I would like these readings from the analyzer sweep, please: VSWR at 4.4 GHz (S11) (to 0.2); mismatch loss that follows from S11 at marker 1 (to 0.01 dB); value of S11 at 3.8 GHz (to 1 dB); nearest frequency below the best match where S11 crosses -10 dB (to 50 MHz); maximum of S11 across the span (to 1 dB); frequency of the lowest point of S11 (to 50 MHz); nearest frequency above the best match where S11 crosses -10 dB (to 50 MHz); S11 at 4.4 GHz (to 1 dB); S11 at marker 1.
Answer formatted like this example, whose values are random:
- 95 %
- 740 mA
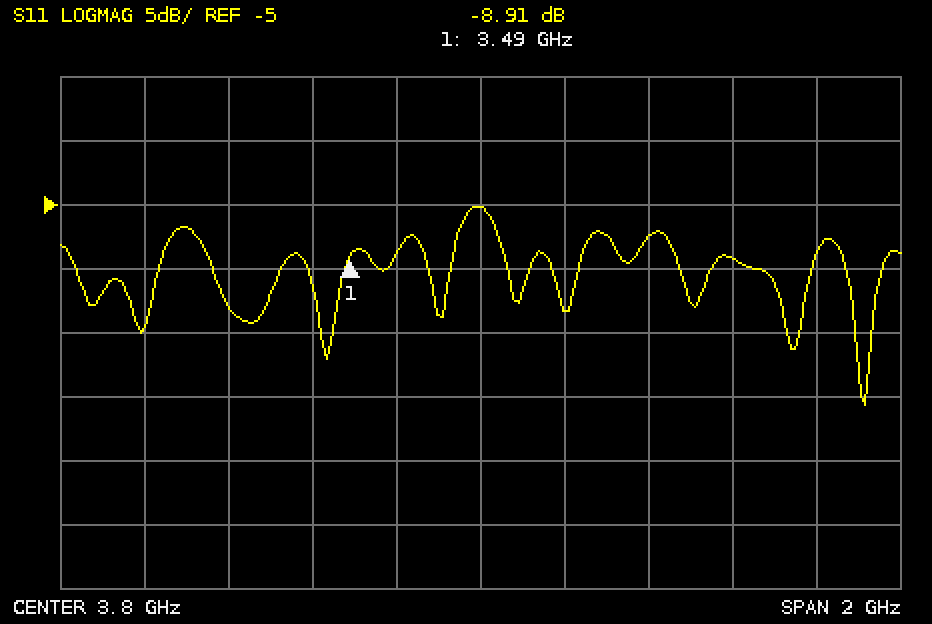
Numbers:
- 2.0
- 0.60 dB
- -5 dB
- 4.65 GHz
- -5 dB
- 4.70 GHz
- 4.75 GHz
- -9 dB
- -8.91 dB
